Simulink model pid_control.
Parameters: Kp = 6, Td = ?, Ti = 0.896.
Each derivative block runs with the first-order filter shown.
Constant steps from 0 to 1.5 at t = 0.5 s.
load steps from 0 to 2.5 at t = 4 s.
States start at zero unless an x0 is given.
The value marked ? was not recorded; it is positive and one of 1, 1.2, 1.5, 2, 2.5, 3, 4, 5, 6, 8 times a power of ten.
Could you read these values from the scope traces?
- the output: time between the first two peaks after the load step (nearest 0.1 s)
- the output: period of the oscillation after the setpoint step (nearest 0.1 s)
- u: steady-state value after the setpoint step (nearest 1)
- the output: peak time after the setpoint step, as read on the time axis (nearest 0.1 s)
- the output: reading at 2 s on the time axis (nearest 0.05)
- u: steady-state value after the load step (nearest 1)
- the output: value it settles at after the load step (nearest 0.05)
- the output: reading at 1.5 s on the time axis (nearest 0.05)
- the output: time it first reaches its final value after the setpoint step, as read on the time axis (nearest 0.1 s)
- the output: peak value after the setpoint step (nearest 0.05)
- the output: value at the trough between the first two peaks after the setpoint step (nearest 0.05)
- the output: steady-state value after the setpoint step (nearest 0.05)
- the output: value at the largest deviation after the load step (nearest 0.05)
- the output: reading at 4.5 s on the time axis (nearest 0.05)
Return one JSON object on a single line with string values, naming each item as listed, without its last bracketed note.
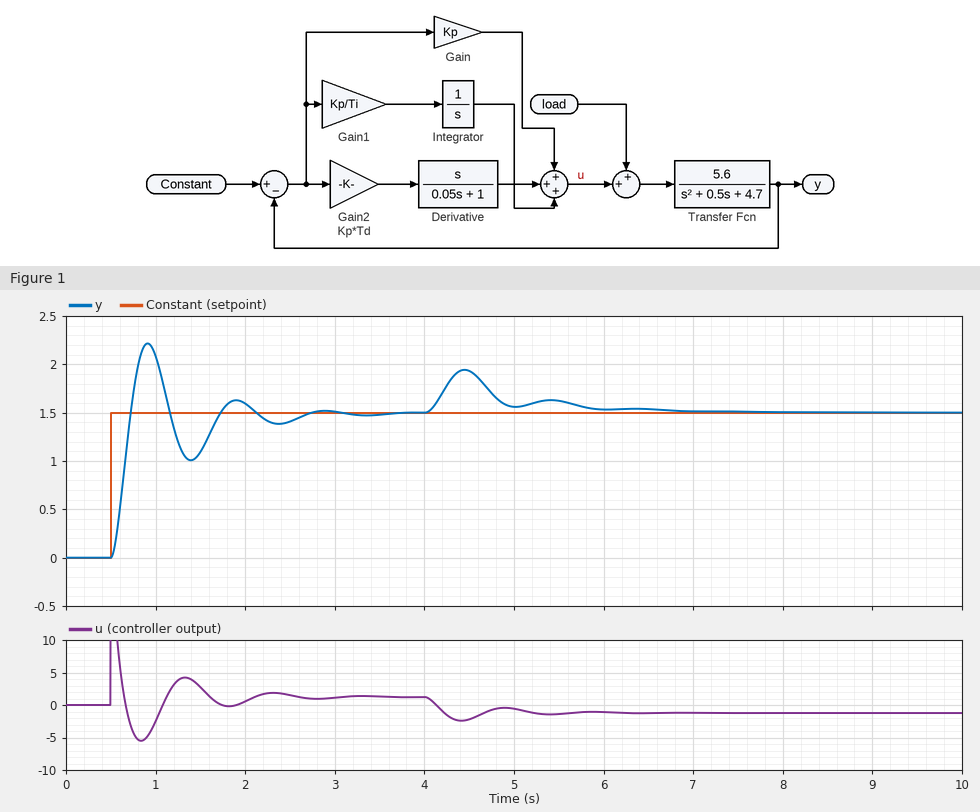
{"the output: time between the first two peaks after the load step": "1.0 s", "the output: period of the oscillation after the setpoint step": "1.0 s", "u: steady-state value after the setpoint step": "1", "the output: peak time after the setpoint step, as read on the time axis": "0.9 s", "the output: reading at 2 s on the time axis": "1.60", "u: steady-state value after the load step": "-1", "the output: value it settles at after the load step": "1.50", "the output: reading at 1.5 s on the time axis": "1.10", "the output: time it first reaches its final value after the setpoint step, as read on the time axis": "0.7 s", "the output: peak value after the setpoint step": "2.20", "the output: value at the trough between the first two peaks after the setpoint step": "1.00", "the output: steady-state value after the setpoint step": "1.50", "the output: value at the largest deviation after the load step": "1.95", "the output: reading at 4.5 s on the time axis": "1.95"}
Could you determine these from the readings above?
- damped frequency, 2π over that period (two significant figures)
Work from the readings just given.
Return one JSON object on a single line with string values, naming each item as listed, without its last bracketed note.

{"damped frequency, 2π over that period": "6.3 rad/s"}
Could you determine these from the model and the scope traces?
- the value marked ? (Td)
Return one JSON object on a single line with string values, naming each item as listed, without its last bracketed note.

{"the value marked ?": "0.1"}
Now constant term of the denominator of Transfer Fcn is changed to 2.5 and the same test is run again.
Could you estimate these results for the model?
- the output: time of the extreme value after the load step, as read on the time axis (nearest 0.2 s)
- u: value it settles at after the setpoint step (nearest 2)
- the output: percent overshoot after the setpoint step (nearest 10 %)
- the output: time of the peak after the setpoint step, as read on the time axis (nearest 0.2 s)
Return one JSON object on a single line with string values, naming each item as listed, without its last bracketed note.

{"the output: time of the extreme value after the load step, as read on the time axis": "4.4 s", "u: value it settles at after the setpoint step": "0", "the output: percent overshoot after the setpoint step": "50 %", "the output: time of the peak after the setpoint step, as read on the time axis": "1.0 s"}
